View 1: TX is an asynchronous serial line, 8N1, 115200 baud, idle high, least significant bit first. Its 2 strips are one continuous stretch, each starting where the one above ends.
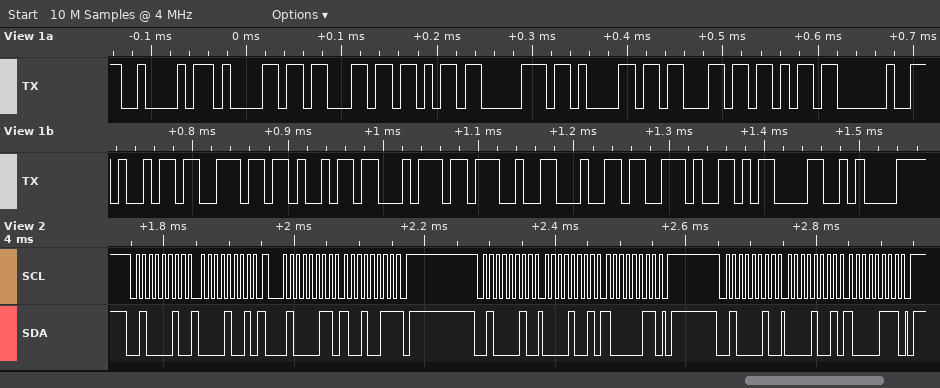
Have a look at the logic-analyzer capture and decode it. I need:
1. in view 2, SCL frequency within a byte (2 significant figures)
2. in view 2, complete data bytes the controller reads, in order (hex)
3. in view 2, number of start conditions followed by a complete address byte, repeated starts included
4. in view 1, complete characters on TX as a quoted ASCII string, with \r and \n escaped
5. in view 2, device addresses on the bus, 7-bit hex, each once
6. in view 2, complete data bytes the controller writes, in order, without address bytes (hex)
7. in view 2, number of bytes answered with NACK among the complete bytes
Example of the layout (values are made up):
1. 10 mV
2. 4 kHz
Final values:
1. 100 kHz
2. 93
3. 4
4. "Backpack init'd.\r\n"
5. 0x21
6. 09 09 83 09 87
7. 1
